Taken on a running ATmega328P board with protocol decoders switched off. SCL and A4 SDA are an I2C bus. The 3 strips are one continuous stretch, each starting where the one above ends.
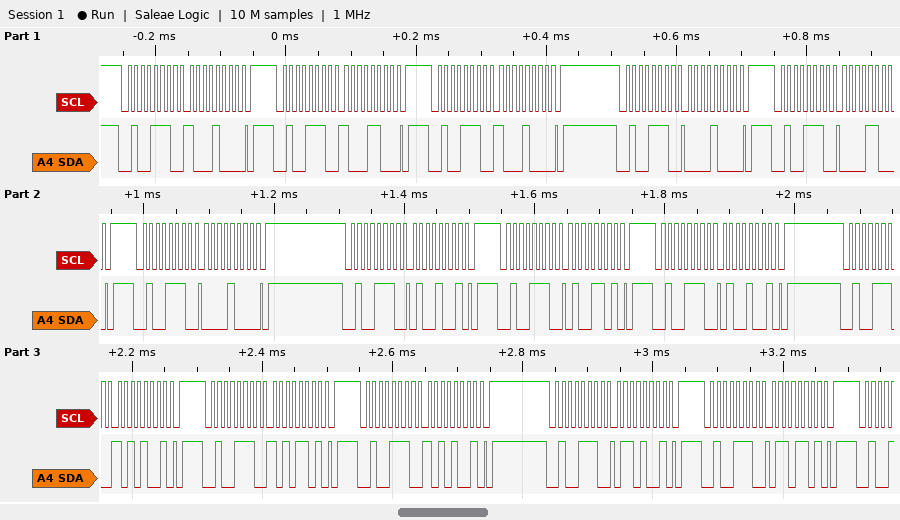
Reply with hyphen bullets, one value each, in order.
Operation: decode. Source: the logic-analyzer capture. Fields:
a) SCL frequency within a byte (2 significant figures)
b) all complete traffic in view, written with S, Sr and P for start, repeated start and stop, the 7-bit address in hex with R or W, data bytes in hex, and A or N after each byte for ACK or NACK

- 100 kHz
- S 27W A 88 A P S 27W A 8C A P S 27W A 88 A P S 27W A 08 A P S 27W A 0C A P S 27W A 08 A P S 27W A 49 A P S 27W A 4D A P S 27W A 49 A P S 27W A A9 A P S 27W A AD A P S 27W A A9 A P S 27W A 69 A P S 27W A 6D A P
